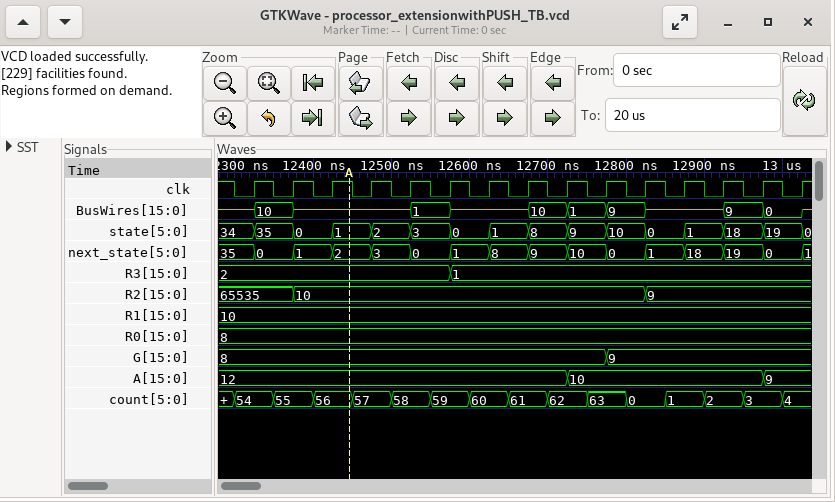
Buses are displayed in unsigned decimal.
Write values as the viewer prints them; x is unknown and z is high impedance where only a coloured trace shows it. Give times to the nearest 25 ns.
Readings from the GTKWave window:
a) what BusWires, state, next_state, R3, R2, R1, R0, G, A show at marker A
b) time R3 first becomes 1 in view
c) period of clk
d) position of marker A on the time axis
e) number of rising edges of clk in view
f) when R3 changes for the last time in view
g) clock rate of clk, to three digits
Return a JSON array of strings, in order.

["BusWires=z, state=1, next_state=2, R3=2, R2=10, R1=10, R0=8, G=8, A=12", "12575 ns", "50 ns", "12450 ns", "15", "12575 ns", "20.0 MHz"]
